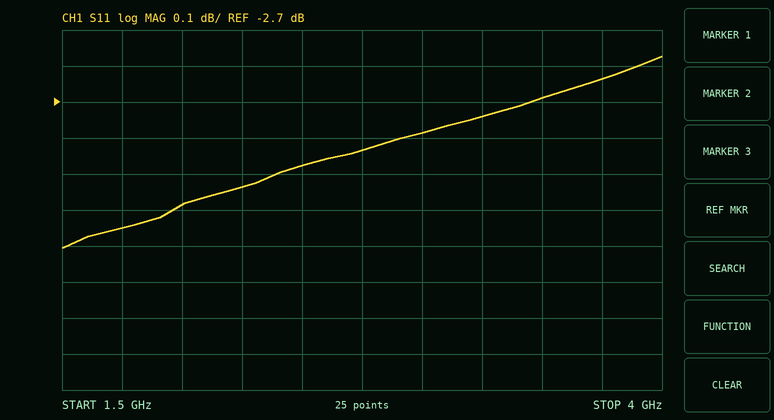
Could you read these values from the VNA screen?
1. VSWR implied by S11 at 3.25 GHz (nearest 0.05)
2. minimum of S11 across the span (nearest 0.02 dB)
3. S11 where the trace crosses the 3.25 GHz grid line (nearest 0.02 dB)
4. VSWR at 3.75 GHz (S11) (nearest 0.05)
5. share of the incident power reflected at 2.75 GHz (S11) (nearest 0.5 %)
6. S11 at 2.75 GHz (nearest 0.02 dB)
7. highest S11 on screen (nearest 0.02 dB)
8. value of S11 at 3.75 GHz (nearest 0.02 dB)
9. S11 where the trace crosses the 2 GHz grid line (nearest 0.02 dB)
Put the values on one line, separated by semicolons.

6.40; -3.10 dB; -2.74 dB; 6.65; 52.0 %; -2.84 dB; -2.58 dB; -2.64 dB; -2.98 dB
